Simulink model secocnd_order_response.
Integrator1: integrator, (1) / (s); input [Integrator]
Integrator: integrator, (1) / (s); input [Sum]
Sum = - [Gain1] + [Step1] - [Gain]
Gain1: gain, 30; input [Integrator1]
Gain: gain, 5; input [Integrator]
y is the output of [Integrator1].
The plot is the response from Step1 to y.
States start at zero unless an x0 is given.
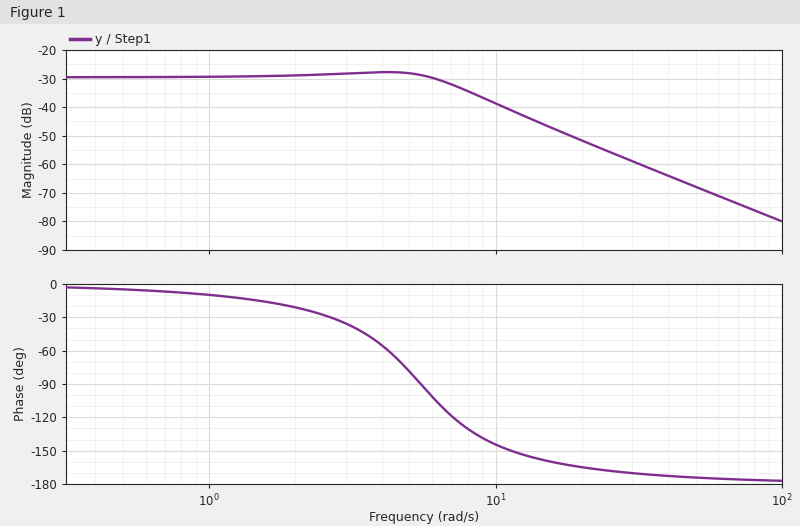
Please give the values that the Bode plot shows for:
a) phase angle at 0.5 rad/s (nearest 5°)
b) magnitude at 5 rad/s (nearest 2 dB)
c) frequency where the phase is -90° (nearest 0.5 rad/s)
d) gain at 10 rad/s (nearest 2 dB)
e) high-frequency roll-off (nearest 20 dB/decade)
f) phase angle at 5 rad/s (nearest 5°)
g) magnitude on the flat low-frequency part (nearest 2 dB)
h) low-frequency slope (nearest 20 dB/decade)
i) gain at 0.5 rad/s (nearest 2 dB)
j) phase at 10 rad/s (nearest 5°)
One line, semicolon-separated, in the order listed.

-5°; -28 dB; 5.5 rad/s; -38 dB; -40 dB/decade; -80°; -30 dB; 0 dB/decade; -30 dB; -145°
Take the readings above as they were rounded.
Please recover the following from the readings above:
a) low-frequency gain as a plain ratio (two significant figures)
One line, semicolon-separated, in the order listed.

0.032
